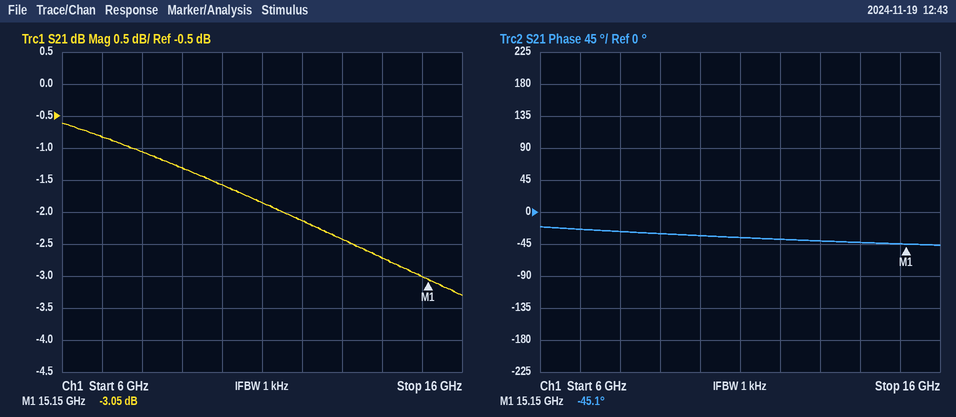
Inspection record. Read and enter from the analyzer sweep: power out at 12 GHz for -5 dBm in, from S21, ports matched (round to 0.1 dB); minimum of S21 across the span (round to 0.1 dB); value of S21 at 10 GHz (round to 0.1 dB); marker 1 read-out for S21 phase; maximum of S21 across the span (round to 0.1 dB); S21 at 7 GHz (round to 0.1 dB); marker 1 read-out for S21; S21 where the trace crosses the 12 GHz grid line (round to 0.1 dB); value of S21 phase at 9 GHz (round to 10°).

-7.1 dBm
-3.3 dB
-1.6 dB
-45.1°
-0.6 dB
-0.8 dB
-3.05 dB
-2.1 dB
-30°
